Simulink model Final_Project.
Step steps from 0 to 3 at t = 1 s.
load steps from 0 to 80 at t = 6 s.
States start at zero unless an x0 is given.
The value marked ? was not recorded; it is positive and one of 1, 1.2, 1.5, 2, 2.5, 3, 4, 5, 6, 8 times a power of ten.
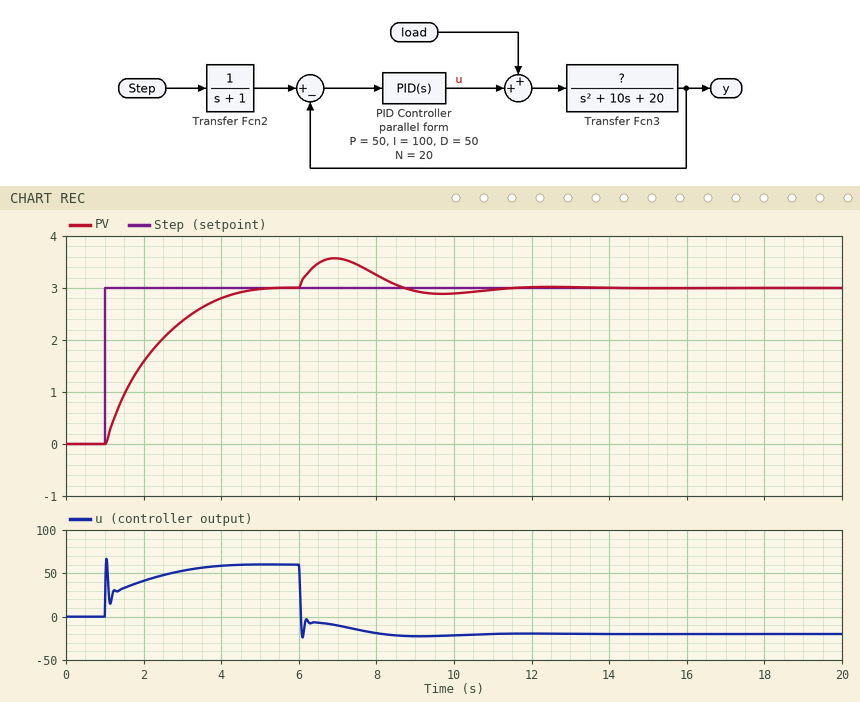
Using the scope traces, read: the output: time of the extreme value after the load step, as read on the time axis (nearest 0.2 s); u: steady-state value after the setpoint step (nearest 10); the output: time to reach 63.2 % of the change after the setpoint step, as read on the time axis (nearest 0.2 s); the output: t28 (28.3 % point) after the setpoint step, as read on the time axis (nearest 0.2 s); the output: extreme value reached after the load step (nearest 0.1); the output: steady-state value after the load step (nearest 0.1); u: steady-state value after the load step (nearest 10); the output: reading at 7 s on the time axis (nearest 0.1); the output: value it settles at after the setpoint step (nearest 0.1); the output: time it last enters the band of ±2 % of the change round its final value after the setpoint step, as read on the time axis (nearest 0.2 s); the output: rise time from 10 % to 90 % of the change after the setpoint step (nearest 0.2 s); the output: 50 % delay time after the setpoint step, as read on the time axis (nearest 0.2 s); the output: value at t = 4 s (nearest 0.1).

7.0 s
60
2.4 s
1.4 s
3.6
3.0
-20
3.6
3.0
4.6 s
2.6 s
2.0 s
2.8
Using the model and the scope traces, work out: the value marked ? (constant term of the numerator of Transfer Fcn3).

1
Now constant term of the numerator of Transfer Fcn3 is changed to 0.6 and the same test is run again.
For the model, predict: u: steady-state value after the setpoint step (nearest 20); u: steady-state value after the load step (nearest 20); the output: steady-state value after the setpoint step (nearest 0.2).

100
20
3.0
